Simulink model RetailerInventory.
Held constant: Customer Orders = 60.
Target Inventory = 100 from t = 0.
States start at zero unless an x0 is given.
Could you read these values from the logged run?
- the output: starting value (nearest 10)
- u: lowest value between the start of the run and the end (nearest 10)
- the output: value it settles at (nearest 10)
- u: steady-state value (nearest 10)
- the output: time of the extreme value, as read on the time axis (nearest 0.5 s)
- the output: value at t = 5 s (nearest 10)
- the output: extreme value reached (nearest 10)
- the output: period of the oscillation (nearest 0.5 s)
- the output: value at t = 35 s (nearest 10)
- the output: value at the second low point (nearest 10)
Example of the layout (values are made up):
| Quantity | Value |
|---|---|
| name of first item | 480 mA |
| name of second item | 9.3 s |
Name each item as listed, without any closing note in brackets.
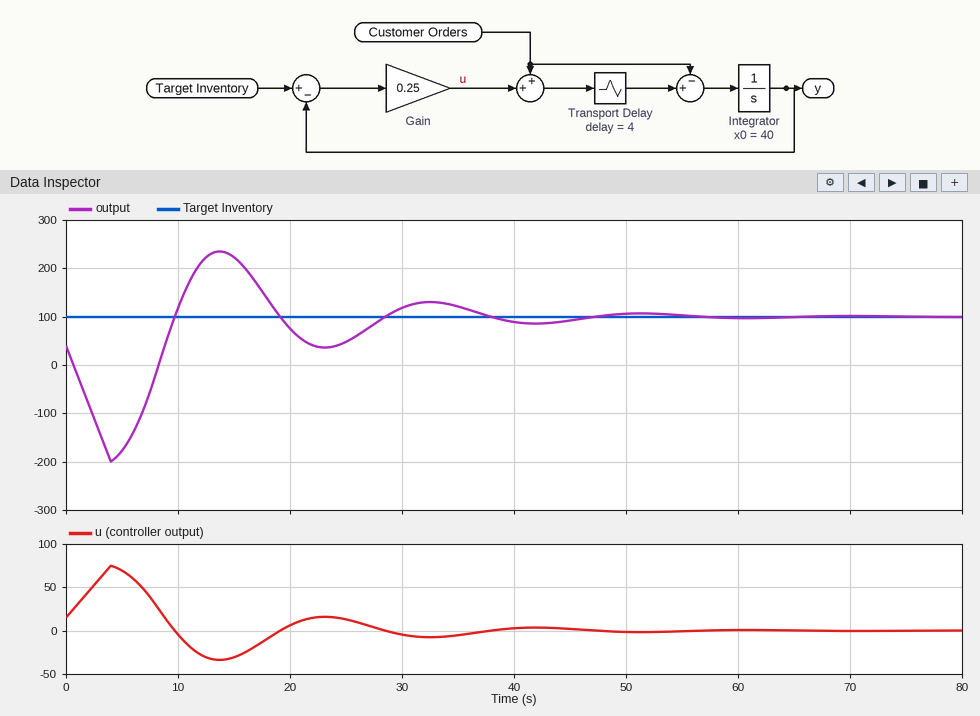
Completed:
| Quantity | Value |
|---|---|
| the output: starting value | 40 |
| u: lowest value between the start of the run and the end | -30 |
| the output: value it settles at | 100 |
| u: steady-state value | 0 |
| the output: time of the extreme value, as read on the time axis | 4.0 s |
| the output: value at t = 5 s | -180 |
| the output: extreme value reached | -200 |
| the output: period of the oscillation | 19.0 s |
| the output: value at t = 35 s | 120 |
| the output: value at the second low point | 40 |
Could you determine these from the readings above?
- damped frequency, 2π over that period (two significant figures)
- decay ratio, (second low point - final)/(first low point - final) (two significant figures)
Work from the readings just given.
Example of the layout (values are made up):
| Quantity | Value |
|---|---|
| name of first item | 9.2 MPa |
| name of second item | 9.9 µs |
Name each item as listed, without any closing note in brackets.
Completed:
| Quantity | Value |
|---|---|
| damped frequency, 2π over that period | 0.33 rad/s |
| decay ratio, (second low point - final)/(first low point - final) | 0.20 |
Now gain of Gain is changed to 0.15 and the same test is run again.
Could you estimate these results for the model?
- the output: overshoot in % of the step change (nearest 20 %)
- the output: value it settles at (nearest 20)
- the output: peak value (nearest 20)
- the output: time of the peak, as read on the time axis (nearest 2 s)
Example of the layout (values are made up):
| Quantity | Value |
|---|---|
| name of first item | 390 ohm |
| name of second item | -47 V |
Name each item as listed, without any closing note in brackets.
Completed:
| Quantity | Value |
|---|---|
| the output: overshoot in % of the step change | 60 % |
| the output: value it settles at | 100 |
| the output: peak value | 140 |
| the output: time of the peak, as read on the time axis | 18 s |
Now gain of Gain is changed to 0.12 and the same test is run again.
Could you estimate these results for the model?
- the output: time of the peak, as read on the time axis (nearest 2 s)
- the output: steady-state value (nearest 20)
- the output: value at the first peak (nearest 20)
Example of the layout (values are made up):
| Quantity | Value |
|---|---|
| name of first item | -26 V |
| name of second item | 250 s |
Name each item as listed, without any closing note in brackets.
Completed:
| Quantity | Value |
|---|---|
| the output: time of the peak, as read on the time axis | 22 s |
| the output: steady-state value | 100 |
| the output: value at the first peak | 100 |
